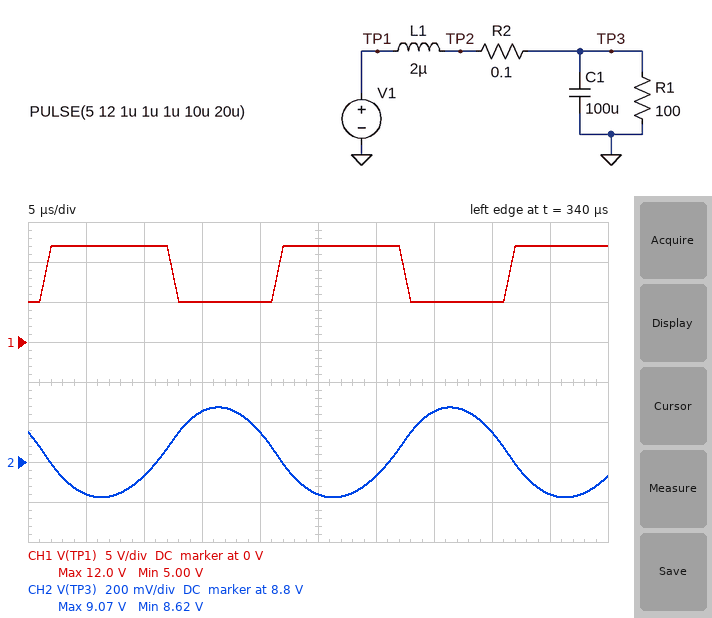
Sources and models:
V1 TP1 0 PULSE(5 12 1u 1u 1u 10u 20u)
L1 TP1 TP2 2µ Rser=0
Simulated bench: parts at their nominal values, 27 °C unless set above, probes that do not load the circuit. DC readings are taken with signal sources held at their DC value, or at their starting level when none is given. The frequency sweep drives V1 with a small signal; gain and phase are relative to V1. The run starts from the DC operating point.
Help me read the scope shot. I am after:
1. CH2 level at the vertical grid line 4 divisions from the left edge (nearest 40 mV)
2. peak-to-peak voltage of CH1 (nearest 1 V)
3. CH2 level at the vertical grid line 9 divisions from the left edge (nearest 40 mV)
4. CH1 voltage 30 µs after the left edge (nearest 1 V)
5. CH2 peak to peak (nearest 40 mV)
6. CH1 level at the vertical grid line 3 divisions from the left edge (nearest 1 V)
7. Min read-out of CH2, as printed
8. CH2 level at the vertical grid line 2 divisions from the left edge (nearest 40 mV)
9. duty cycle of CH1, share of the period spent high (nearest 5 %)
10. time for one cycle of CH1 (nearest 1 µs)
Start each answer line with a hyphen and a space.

- 8.96 V
- 7 V
- 8.64 V
- 12 V
- 440 mV
- 5 V
- 8.62 V
- 8.72 V
- 55 %
- 20 µs
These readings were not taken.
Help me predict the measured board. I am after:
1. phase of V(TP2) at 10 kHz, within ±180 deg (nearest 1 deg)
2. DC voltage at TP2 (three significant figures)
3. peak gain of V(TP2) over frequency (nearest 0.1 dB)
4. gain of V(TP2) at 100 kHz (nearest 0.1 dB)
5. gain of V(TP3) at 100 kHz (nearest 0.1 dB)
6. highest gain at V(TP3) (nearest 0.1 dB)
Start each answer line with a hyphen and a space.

- -39 deg
- 5.00 V
- 5.0 dB
- -21.8 dB
- -37.9 dB
- 3.6 dB
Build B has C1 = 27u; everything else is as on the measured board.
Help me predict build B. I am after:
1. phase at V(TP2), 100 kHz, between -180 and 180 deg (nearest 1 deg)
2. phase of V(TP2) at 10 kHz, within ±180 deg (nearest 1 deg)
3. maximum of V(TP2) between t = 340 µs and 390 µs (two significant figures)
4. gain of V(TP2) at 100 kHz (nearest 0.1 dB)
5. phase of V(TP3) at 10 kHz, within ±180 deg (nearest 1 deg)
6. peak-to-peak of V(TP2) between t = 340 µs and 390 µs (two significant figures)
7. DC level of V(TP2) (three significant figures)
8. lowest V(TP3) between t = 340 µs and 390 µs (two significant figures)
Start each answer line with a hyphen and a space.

- -116 deg
- -3 deg
- 10 V
- -20.3 dB
- -12 deg
- 2.6 V
- 5.00 V
- 7.9 V
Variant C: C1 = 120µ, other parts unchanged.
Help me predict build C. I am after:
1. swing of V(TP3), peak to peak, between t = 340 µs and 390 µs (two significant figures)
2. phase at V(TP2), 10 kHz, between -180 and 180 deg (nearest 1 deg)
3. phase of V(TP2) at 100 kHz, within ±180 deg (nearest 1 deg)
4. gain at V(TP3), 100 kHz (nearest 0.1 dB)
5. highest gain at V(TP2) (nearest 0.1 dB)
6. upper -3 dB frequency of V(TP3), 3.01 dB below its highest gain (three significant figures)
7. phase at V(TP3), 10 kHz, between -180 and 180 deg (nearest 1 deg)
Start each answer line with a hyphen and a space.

- 370 mV
- -49 deg
- -93 deg
- -39.5 dB
- 4.5 dB
- 12.2 kHz
- -86 deg
